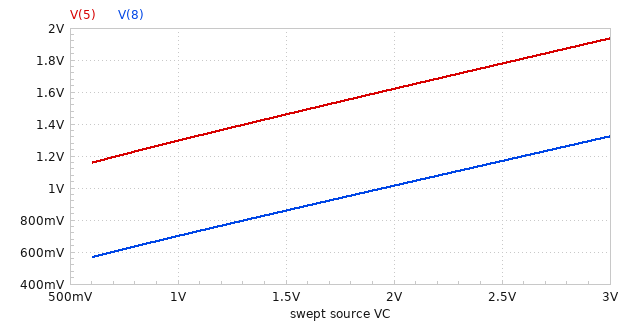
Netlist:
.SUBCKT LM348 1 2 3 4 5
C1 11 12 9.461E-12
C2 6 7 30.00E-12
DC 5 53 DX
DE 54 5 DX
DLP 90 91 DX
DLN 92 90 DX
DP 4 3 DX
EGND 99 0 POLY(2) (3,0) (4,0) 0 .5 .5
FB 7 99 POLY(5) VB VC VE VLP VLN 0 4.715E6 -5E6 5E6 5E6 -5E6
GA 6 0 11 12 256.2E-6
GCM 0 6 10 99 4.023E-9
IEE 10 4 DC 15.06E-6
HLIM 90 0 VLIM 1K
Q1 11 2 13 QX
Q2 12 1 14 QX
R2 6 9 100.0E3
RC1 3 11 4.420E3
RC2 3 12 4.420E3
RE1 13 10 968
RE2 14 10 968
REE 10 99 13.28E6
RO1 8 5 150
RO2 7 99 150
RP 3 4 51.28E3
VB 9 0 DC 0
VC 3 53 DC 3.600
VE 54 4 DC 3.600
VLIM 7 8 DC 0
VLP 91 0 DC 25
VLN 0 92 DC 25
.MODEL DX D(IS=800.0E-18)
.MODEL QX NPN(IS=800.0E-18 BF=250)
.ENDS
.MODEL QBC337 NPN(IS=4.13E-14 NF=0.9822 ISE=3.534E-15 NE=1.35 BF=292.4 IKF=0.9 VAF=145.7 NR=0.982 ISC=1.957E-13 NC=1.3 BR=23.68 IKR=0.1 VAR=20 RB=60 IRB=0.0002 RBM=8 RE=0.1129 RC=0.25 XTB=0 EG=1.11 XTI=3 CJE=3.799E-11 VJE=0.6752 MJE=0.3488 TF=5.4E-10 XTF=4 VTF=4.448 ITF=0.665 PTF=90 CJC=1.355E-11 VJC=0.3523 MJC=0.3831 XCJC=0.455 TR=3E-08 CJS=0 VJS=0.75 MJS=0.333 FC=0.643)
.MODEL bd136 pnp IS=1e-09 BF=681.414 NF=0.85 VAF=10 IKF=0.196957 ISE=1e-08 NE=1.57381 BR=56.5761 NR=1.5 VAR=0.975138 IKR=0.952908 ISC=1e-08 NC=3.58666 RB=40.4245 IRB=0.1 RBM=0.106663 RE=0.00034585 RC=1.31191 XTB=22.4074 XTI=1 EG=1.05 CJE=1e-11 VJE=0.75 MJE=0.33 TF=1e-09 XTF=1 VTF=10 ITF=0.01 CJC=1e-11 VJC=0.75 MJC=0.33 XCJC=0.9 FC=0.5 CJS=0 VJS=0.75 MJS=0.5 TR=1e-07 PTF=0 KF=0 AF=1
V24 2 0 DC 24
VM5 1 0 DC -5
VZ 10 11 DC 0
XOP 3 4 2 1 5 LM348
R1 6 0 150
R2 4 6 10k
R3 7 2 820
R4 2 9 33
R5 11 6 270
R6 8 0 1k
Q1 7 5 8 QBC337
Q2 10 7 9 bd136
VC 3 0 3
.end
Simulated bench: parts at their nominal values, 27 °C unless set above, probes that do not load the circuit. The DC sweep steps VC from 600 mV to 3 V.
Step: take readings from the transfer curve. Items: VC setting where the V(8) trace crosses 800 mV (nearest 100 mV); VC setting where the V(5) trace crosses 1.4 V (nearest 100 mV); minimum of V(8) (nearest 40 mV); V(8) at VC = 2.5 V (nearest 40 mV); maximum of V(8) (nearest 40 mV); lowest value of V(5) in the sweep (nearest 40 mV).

1.3 V
1.3 V
560 mV
1.16 V
1.32 V
1.16 V
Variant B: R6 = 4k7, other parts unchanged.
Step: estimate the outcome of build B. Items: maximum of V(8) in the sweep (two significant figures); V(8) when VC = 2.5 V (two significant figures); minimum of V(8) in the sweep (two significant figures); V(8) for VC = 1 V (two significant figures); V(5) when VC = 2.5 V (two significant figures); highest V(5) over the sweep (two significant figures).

6.2 V
5.5 V
2.7 V
3.3 V
6.1 V
6.8 V
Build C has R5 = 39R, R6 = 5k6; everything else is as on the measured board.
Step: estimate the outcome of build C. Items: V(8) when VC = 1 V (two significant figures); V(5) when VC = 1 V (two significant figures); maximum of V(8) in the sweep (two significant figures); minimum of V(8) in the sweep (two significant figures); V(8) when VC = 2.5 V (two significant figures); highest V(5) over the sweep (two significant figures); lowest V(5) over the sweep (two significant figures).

3.9 V
4.5 V
7.3 V
3.2 V
6.5 V
7.9 V
3.8 V
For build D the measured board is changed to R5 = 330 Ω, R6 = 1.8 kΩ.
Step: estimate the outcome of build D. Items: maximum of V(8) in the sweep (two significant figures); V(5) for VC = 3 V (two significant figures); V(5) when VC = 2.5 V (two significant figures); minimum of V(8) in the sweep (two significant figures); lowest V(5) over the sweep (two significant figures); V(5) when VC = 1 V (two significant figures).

2.4 V
3.0 V
2.7 V
1.0 V
1.6 V
1.9 V
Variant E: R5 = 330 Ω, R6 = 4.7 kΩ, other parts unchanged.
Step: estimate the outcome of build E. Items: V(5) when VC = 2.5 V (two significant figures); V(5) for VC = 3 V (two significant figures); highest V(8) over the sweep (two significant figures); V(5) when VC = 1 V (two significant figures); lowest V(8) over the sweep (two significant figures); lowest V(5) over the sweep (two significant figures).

6.1 V
6.9 V
6.2 V
3.9 V
2.7 V
3.3 V
